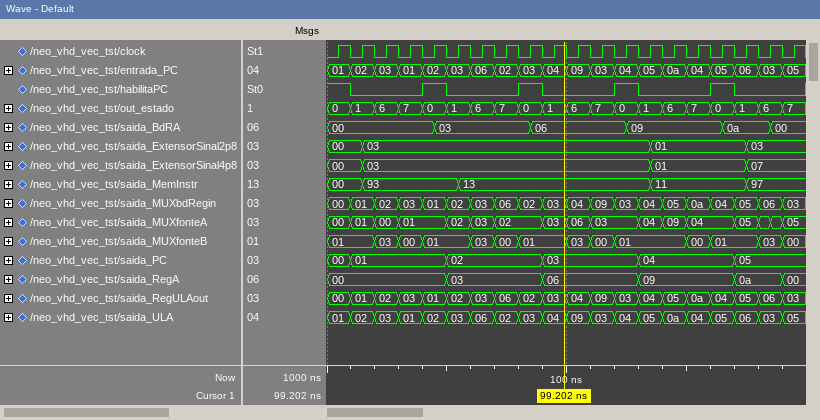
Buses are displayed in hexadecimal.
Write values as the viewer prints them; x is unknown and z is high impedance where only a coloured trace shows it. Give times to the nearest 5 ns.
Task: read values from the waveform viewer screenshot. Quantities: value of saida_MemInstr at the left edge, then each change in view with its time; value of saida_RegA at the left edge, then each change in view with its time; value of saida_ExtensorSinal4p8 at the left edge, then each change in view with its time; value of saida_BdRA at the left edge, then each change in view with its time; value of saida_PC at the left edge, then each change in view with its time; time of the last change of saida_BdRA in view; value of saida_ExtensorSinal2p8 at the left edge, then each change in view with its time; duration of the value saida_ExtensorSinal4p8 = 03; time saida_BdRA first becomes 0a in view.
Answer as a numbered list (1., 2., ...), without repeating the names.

1. 00, 93 at 15 ns, 13 at 55 ns, 11 at 135 ns, 97 at 175 ns
2. 00, 03 at 50 ns, 06 at 90 ns, 09 at 130 ns, 0a at 170 ns, 00 at 190 ns
3. 00, 03 at 15 ns, 01 at 135 ns, 07 at 175 ns
4. 00, 03 at 45 ns, 06 at 85 ns, 09 at 125 ns, 0a at 165 ns, 00 at 185 ns
5. 00, 01 at 10 ns, 02 at 50 ns, 03 at 90 ns, 04 at 130 ns, 05 at 170 ns
6. 185 ns
7. 00, 03 at 15 ns, 01 at 135 ns, 03 at 175 ns
8. 120 ns
9. 165 ns
